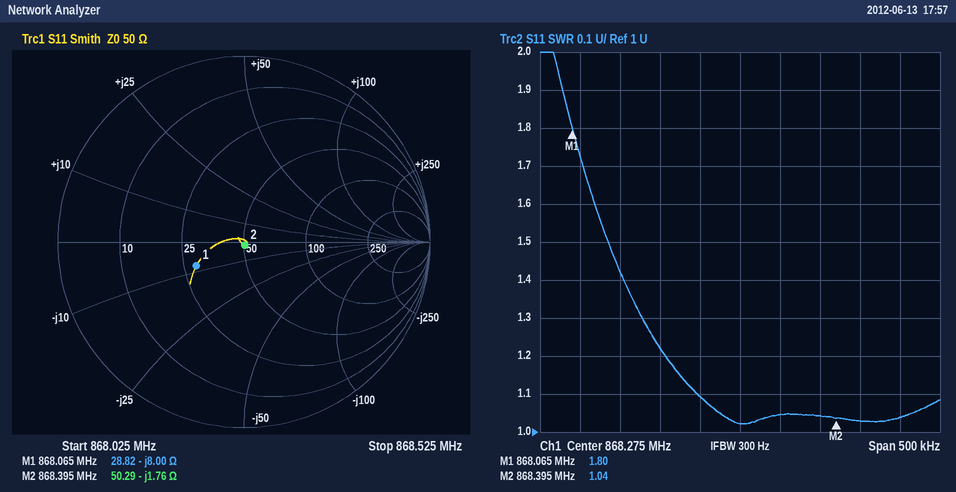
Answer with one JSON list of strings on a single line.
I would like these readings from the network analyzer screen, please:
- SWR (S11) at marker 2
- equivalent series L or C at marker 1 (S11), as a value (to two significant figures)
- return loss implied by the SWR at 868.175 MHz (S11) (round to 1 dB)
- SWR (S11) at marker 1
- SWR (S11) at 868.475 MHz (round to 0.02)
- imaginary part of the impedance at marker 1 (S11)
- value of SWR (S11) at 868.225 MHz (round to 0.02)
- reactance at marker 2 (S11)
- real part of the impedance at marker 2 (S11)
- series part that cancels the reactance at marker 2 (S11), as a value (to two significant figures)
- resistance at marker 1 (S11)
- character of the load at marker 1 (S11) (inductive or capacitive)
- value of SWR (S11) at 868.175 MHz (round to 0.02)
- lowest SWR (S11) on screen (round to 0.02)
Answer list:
["1.04", "23 pF", "20 dB", "1.80", "1.04", "-8.00 Ω", "1.10", "-1.76 Ω", "50.29 Ω", "320 pH", "28.82 Ω", "capacitive", "1.22", "1.02"]
